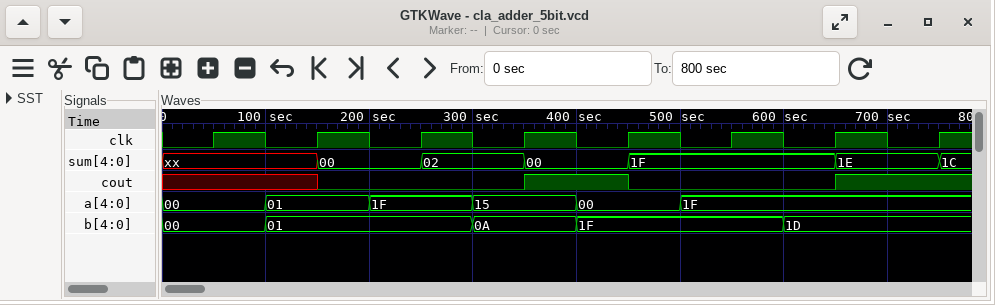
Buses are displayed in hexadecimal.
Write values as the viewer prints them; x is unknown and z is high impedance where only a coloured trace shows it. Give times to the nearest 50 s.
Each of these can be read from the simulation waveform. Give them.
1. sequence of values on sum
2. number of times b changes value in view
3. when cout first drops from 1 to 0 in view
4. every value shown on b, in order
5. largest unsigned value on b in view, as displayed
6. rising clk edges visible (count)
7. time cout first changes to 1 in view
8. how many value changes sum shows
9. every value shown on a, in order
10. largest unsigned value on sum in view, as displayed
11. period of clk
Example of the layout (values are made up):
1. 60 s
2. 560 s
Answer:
1. xx, 00, 02, 00, 1F, 1E, 1C
2. 4
3. 450 s
4. 00, 01, 0A, 1F, 1D
5. 1F
6. 8
7. 350 s
8. 6
9. 00, 01, 1F, 15, 00, 1F
10. 1F
11. 100 s
